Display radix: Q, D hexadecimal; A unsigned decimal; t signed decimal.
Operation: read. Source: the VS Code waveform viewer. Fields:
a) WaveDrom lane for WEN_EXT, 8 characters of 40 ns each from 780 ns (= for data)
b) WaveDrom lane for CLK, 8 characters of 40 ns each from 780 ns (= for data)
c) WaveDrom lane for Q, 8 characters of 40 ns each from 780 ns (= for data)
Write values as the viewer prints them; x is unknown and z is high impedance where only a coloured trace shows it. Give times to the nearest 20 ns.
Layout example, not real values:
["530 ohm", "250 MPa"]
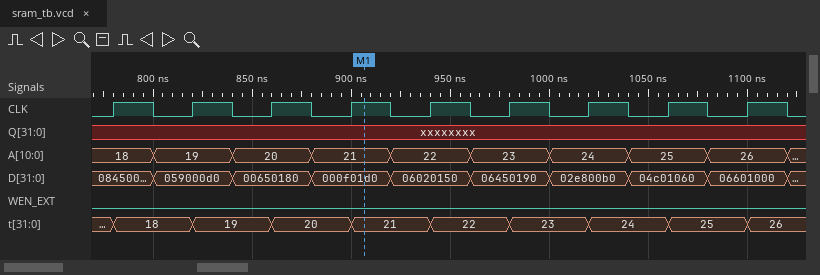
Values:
["{name: 'WEN_EXT', wave: '0.......'}", "{name: 'CLK', wave: 'p.......'}", "{name: 'Q', wave: 'x.......'}"]
